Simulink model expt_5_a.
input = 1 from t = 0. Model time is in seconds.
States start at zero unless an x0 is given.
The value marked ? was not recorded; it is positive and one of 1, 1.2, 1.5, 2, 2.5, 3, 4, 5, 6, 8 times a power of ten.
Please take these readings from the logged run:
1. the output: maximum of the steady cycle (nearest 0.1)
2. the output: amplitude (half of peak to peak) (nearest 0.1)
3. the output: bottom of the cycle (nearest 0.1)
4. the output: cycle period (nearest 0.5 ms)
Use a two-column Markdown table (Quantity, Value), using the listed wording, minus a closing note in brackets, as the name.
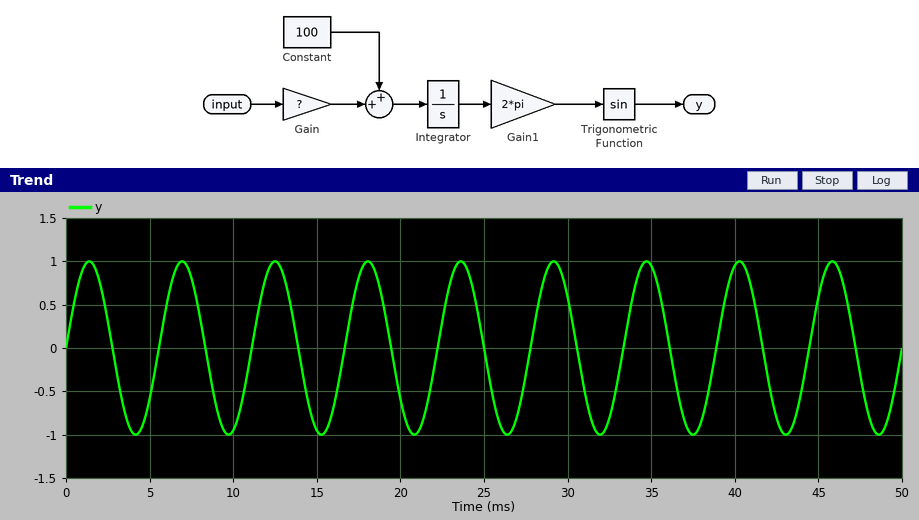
| Quantity | Value |
|---|---|
| the output: maximum of the steady cycle | 1.0 |
| the output: amplitude (half of peak to peak) | 1.0 |
| the output: bottom of the cycle | -1.0 |
| the output: cycle period | 5.5 ms |
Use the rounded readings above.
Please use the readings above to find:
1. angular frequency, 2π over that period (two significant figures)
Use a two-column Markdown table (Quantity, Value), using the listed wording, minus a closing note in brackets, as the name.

| Quantity | Value |
|---|---|
| angular frequency, 2π over that period | 1.1 rad/ms |
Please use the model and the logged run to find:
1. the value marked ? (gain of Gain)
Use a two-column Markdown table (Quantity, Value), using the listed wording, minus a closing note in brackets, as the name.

| Quantity | Value |
|---|---|
| the value marked ? | 80 |
